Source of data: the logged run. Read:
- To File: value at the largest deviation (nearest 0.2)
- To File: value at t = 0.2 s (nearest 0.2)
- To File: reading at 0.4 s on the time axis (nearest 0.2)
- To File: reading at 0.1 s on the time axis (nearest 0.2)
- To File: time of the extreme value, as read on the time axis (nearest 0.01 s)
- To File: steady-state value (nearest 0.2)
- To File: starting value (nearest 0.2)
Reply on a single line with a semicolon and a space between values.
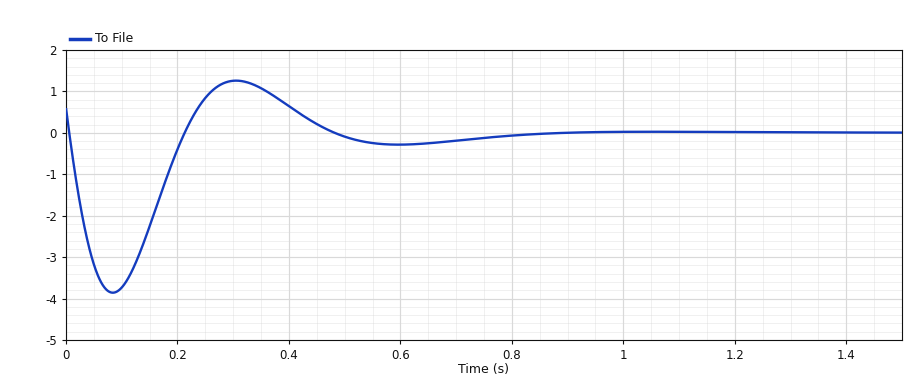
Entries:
-3.8; -0.4; 0.6; -3.8; 0.08 s; 0.0; 0.6
